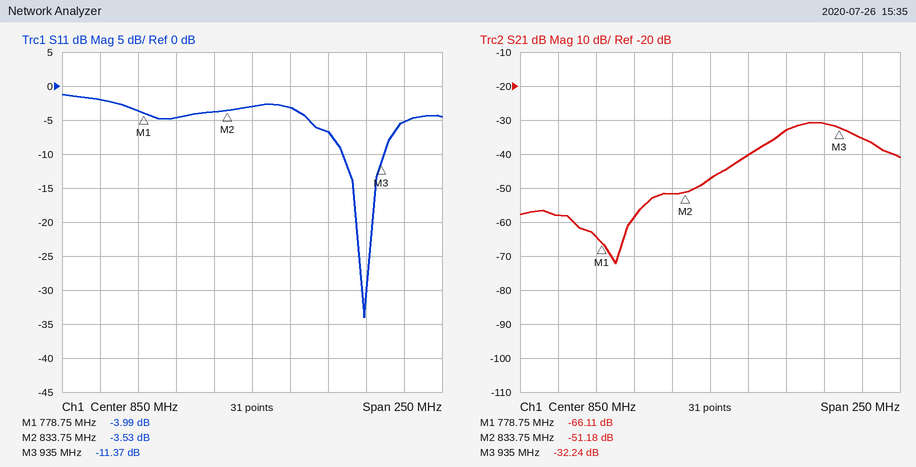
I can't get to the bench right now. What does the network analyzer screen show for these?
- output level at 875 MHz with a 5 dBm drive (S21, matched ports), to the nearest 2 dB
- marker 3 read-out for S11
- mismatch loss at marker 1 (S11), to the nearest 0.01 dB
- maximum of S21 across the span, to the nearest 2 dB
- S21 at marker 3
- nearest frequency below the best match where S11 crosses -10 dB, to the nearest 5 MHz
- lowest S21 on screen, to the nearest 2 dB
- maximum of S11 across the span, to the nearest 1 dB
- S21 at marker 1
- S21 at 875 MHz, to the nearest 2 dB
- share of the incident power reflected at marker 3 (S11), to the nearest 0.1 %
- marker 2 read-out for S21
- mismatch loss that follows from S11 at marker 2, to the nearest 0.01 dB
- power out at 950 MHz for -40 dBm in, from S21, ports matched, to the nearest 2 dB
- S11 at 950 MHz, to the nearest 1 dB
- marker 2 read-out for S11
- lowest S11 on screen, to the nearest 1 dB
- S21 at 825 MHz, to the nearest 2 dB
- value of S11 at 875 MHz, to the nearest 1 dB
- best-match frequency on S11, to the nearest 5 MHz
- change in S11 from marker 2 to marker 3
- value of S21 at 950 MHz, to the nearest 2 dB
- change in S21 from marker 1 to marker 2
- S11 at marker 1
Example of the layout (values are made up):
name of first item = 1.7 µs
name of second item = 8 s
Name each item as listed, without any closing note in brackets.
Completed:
output level at 875 MHz with a 5 dBm drive (S21, matched ports), to the nearest 2 dB = -36 dBm
marker 3 read-out for S11 = -11.37 dB
mismatch loss at marker 1 (S11), to the nearest 0.01 dB = 2.21 dB
maximum of S21 across the span, to the nearest 2 dB = -30 dB
S21 at marker 3 = -32.24 dB
nearest frequency below the best match where S11 crosses -10 dB, to the nearest 5 MHz = 910 MHz
lowest S21 on screen, to the nearest 2 dB = -72 dB
maximum of S11 across the span, to the nearest 1 dB = -1 dB
S21 at marker 1 = -66.11 dB
S21 at 875 MHz, to the nearest 2 dB = -40 dB
share of the incident power reflected at marker 3 (S11), to the nearest 0.1 % = 7.3 %
marker 2 read-out for S21 = -51.18 dB
mismatch loss that follows from S11 at marker 2, to the nearest 0.01 dB = 2.55 dB
power out at 950 MHz for -40 dBm in, from S21, ports matched, to the nearest 2 dB = -76 dBm
S11 at 950 MHz, to the nearest 1 dB = -5 dB
marker 2 read-out for S11 = -3.53 dB
lowest S11 on screen, to the nearest 1 dB = -34 dB
S21 at 825 MHz, to the nearest 2 dB = -52 dB
value of S11 at 875 MHz, to the nearest 1 dB = -3 dB
best-match frequency on S11, to the nearest 5 MHz = 925 MHz
change in S11 from marker 2 to marker 3 = -7.84 dB
value of S21 at 950 MHz, to the nearest 2 dB = -36 dB
change in S21 from marker 1 to marker 2 = 14.93 dB
S11 at marker 1 = -3.99 dB
